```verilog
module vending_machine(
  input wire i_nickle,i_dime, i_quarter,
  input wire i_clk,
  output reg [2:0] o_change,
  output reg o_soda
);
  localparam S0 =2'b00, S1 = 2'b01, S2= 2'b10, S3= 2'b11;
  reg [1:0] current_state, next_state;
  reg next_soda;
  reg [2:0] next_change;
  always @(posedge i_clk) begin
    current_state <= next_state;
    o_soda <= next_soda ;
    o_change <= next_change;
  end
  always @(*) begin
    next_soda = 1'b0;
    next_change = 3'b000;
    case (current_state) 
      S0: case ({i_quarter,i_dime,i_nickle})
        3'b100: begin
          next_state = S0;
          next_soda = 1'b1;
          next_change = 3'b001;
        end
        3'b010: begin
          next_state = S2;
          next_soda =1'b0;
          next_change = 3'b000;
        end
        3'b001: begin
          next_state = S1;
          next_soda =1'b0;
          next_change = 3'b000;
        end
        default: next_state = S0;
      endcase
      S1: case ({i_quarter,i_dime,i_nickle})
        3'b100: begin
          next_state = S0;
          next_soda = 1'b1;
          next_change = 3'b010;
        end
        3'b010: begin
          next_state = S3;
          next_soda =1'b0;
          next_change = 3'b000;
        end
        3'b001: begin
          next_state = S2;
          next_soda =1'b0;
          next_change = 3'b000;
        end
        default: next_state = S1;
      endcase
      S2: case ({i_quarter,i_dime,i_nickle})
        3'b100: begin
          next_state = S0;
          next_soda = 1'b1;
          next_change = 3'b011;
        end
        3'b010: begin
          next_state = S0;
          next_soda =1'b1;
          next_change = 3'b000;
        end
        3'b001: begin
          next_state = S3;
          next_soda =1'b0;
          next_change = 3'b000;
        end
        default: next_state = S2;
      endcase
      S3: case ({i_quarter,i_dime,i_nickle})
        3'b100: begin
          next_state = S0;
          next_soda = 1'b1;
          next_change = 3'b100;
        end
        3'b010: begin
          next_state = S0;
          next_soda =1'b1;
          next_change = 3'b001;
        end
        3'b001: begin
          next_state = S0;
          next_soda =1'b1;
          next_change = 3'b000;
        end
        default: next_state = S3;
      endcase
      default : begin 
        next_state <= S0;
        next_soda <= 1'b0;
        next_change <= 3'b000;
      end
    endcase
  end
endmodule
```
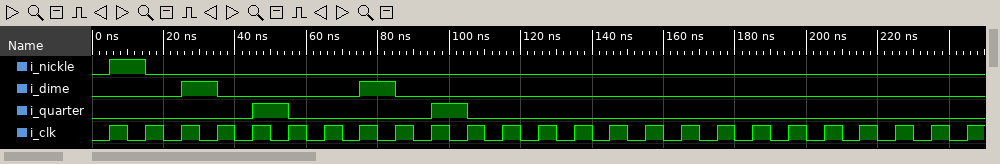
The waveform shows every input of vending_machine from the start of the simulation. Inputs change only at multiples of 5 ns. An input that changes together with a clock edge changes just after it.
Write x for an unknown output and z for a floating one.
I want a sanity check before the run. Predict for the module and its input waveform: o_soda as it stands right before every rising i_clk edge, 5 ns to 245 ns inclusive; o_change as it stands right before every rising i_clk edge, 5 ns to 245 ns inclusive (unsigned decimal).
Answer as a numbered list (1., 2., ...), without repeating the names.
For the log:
1. x 0 0 0 0 0 1 0 0 0 0 1 0 0 0 0 0 0 0 0 0 0 0 0 0
2. x, 0, 0, 0, 0, 0, 4, 0, 0, 0, 0, 3, 0, 0, 0, 0, 0, 0, 0, 0, 0, 0, 0, 0, 0
